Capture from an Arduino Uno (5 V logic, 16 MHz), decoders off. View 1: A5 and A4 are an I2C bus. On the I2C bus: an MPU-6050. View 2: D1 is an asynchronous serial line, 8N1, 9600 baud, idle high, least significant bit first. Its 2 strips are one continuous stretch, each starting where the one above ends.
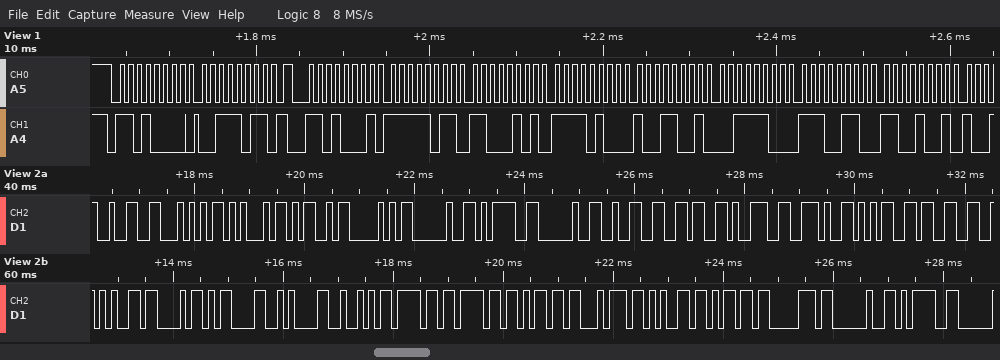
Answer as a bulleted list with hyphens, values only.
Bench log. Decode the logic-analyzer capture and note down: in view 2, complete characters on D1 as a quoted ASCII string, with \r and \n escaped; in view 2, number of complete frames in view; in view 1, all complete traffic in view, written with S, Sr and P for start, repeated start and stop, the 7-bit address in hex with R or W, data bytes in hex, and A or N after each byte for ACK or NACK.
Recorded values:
- "2TEMP = 269.53*C\r\nRoomtemp ="
- 28
- S 68W A 3B A Sr 68R A FB A C5 A F4 A 99 A 3C A E6 A C9 A
